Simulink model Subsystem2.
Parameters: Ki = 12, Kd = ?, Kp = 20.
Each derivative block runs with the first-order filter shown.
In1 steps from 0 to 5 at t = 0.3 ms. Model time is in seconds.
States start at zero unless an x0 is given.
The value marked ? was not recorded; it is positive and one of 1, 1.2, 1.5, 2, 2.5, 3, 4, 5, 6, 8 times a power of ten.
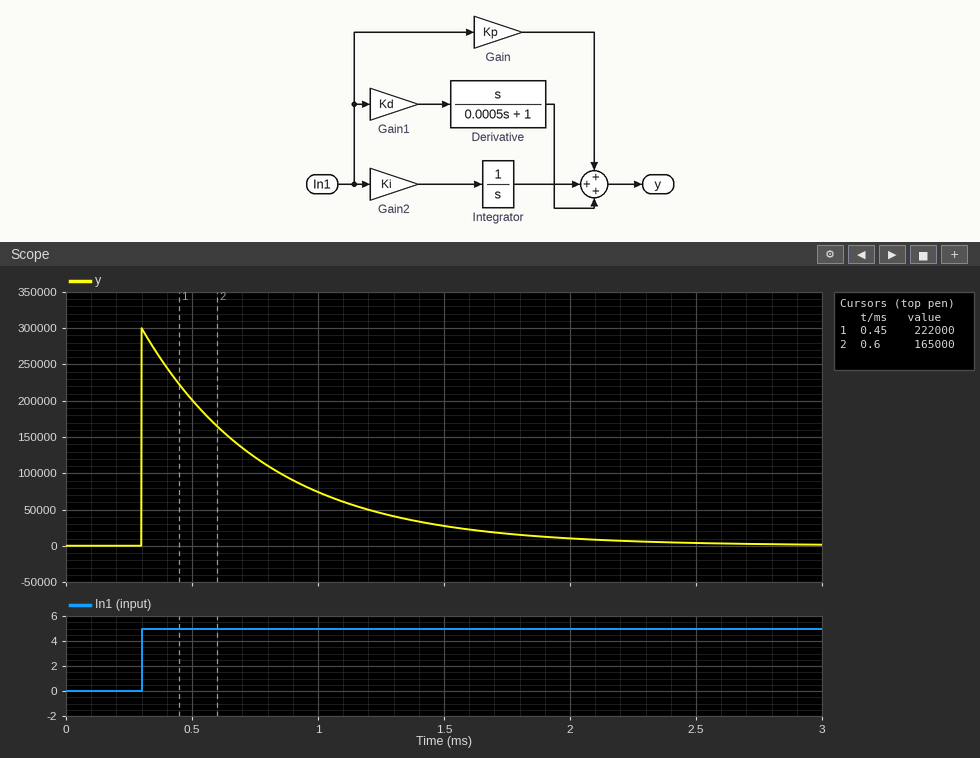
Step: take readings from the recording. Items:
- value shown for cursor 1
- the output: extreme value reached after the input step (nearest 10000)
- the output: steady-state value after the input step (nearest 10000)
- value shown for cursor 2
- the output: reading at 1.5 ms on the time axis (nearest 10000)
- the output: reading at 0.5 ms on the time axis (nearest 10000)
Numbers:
222000
300000
0
165000
30000
200000
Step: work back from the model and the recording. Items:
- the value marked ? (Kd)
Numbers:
30
